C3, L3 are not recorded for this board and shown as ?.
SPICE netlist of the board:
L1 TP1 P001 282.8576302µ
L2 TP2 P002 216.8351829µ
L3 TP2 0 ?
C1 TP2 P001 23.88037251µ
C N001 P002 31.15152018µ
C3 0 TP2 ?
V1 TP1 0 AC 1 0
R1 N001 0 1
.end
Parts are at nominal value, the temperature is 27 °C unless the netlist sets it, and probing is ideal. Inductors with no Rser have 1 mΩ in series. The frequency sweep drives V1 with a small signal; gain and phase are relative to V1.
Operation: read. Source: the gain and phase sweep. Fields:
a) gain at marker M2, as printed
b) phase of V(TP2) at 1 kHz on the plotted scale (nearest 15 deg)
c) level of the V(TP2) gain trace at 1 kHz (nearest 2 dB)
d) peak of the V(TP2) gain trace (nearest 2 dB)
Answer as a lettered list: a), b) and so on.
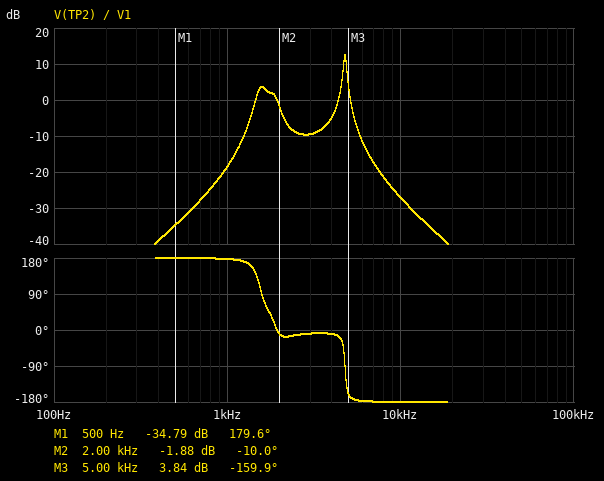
a) -1.88 dB
b) 180 deg
c) -18 dB
d) 12 dB
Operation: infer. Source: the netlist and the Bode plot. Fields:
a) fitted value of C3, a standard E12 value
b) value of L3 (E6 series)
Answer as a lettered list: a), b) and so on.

a) 27 µF
b) 68 µH
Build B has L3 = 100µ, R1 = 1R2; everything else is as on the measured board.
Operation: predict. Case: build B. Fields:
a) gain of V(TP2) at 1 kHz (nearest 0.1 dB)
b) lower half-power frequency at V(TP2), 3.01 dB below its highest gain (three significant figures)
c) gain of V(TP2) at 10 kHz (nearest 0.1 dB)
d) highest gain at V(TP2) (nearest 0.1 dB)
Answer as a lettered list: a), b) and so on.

a) -13.6 dB
b) 4.18 kHz
c) -27.6 dB
d) 10.1 dB
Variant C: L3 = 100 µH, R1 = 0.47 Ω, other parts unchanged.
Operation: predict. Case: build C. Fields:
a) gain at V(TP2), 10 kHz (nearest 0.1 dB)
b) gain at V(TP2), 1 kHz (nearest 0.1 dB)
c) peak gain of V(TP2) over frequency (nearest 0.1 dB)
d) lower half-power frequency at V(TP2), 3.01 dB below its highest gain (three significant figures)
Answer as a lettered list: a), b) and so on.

a) -27.6 dB
b) -13.4 dB
c) 17.8 dB
d) 4.29 kHz
